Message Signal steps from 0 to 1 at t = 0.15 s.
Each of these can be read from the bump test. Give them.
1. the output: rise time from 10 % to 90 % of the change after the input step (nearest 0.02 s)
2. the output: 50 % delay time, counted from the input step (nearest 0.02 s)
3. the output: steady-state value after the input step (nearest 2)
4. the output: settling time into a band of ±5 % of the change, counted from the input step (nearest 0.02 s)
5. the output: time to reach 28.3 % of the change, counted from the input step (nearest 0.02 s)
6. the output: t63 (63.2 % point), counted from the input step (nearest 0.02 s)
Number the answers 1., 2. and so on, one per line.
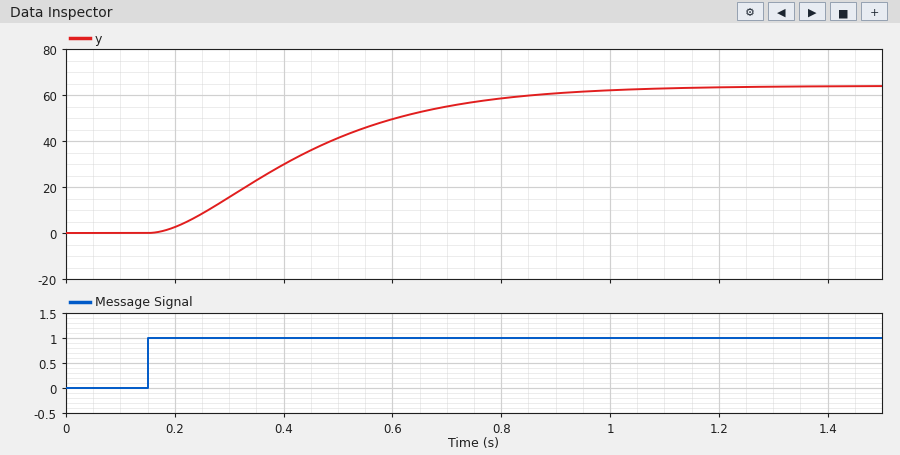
1. 0.54 s
2. 0.26 s
3. 64
4. 0.76 s
5. 0.16 s
6. 0.34 s
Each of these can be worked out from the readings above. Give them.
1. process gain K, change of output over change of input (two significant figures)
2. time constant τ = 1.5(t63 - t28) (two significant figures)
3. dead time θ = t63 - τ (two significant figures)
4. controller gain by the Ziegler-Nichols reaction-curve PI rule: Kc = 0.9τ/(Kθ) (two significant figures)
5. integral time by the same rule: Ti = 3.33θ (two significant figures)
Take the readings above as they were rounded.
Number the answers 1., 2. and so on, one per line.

1. 64
2. 0.27 s
3. 0.070 s
4. 0.054
5. 0.23 s
